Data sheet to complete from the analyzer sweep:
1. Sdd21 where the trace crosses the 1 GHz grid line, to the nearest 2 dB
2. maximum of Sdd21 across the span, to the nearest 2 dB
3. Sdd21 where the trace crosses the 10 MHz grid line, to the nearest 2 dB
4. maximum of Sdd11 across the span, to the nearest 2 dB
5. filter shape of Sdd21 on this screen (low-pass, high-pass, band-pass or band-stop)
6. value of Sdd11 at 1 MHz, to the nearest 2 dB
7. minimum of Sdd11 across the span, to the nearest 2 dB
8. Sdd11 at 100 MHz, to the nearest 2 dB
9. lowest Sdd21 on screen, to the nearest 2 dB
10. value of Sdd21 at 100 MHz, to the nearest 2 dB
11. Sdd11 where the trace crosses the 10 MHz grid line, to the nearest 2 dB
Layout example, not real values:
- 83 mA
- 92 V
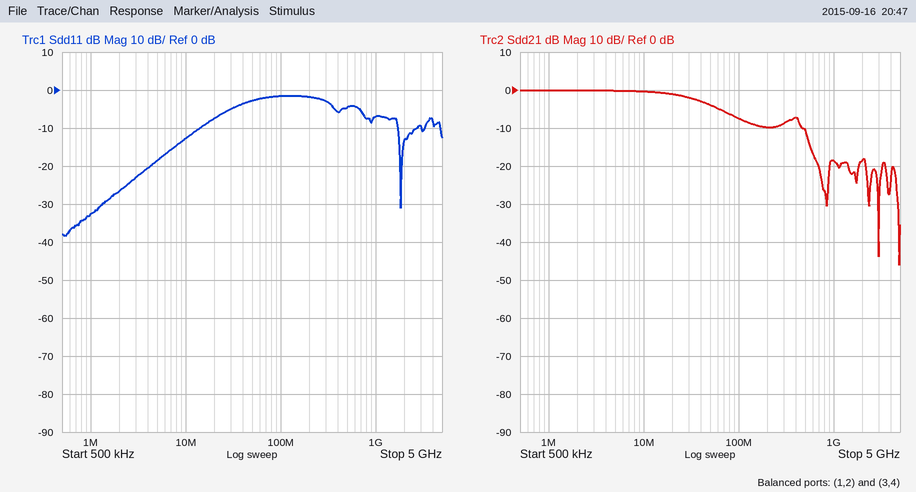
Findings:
- -18 dB
- 0 dB
- 0 dB
- -2 dB
- low-pass
- -32 dB
- -38 dB
- -2 dB
- -46 dB
- -8 dB
- -12 dB
